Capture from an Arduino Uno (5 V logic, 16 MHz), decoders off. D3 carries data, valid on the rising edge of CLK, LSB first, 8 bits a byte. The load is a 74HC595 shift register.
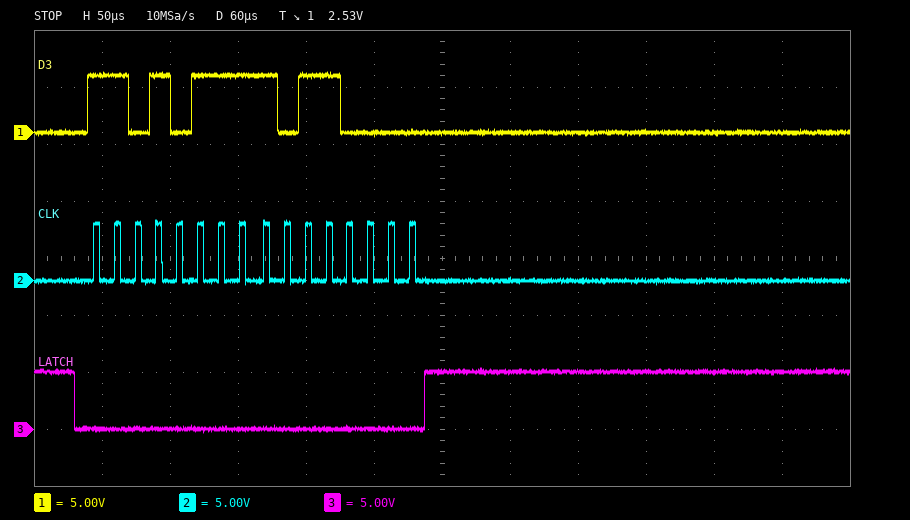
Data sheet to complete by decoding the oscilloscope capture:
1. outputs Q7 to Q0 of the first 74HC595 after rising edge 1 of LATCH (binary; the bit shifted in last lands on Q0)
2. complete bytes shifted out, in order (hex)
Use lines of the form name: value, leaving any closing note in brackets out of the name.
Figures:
outputs Q7 to Q0 of the first 74HC595 after rising edge 1 of LATCH: 10110000
complete bytes shifted out, in order: EB 0D
